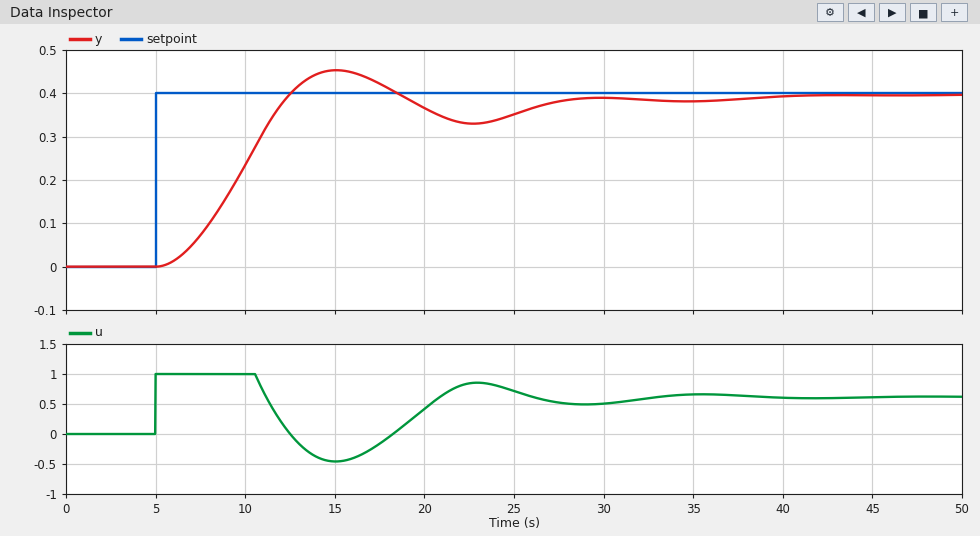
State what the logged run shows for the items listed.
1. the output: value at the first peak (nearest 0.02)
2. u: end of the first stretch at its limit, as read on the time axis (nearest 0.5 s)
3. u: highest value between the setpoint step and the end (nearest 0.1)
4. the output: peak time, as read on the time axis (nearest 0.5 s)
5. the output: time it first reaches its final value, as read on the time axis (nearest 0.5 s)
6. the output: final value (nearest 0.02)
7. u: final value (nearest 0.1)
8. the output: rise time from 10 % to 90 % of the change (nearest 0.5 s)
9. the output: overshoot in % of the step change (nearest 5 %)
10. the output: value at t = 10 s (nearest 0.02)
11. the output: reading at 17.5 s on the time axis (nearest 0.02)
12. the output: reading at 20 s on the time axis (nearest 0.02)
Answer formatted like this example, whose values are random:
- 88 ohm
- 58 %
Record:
- 0.46
- 10.5 s
- 1.0
- 15.0 s
- 12.5 s
- 0.40
- 0.6
- 5.0 s
- 15 %
- 0.24
- 0.42
- 0.36
